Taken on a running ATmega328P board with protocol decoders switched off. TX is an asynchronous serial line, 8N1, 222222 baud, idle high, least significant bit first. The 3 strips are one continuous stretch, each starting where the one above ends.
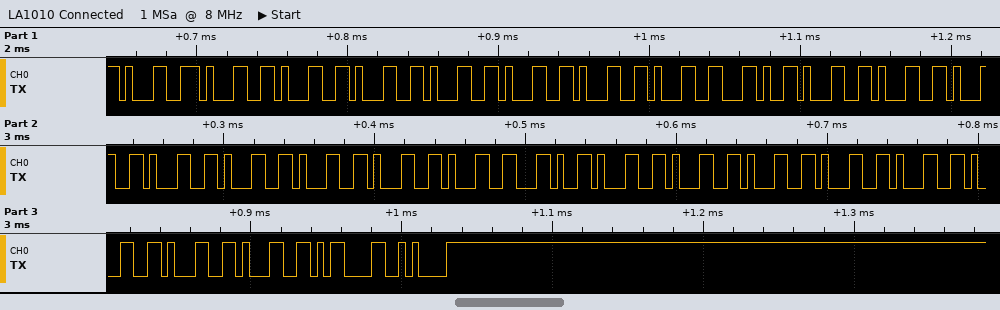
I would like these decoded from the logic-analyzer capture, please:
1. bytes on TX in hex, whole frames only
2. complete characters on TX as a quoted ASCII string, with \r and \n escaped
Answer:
31 31 31 31 31 31 31 31 2C 31 31 31 31 31 31 31 31 2C 31 31 31 31 31 31 31 31 0D 0A
"11111111,11111111,11111111\r\n"
